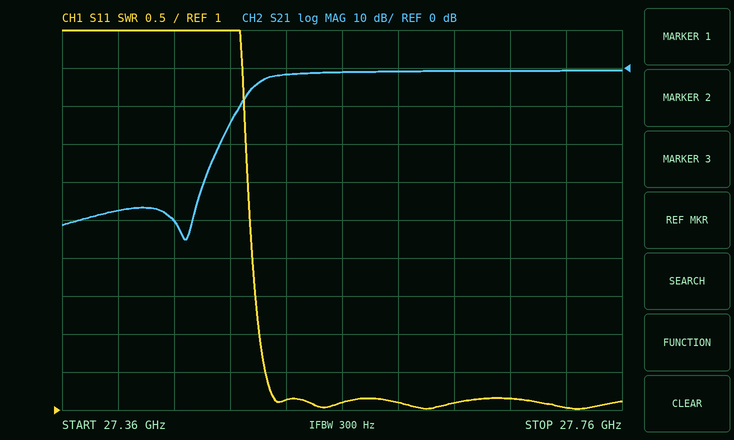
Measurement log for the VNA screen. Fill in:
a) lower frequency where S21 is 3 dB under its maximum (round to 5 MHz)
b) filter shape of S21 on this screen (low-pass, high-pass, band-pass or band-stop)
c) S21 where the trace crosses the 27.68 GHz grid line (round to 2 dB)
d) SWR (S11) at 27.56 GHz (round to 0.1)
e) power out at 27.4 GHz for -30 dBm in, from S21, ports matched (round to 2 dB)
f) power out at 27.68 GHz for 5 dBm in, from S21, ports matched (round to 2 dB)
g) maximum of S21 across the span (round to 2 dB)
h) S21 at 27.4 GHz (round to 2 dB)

27.500 GHz
high-pass
0 dB
1.1
-68 dBm
4 dBm
0 dB
-38 dB
